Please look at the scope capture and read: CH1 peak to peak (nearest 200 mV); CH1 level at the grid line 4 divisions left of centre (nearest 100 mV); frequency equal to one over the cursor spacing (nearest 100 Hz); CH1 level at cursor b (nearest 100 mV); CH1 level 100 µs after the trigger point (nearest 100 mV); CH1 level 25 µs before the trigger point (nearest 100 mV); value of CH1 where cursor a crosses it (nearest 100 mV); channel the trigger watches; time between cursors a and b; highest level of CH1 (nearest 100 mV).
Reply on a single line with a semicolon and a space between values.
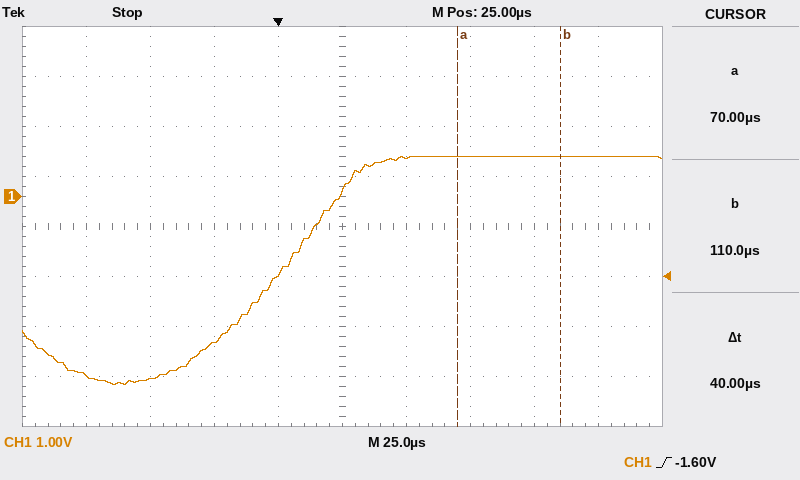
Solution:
4.6 V; -3.6 V; 25.0 kHz; 800 mV; 800 mV; -2.9 V; 800 mV; CH1; 40 µs; 800 mV
